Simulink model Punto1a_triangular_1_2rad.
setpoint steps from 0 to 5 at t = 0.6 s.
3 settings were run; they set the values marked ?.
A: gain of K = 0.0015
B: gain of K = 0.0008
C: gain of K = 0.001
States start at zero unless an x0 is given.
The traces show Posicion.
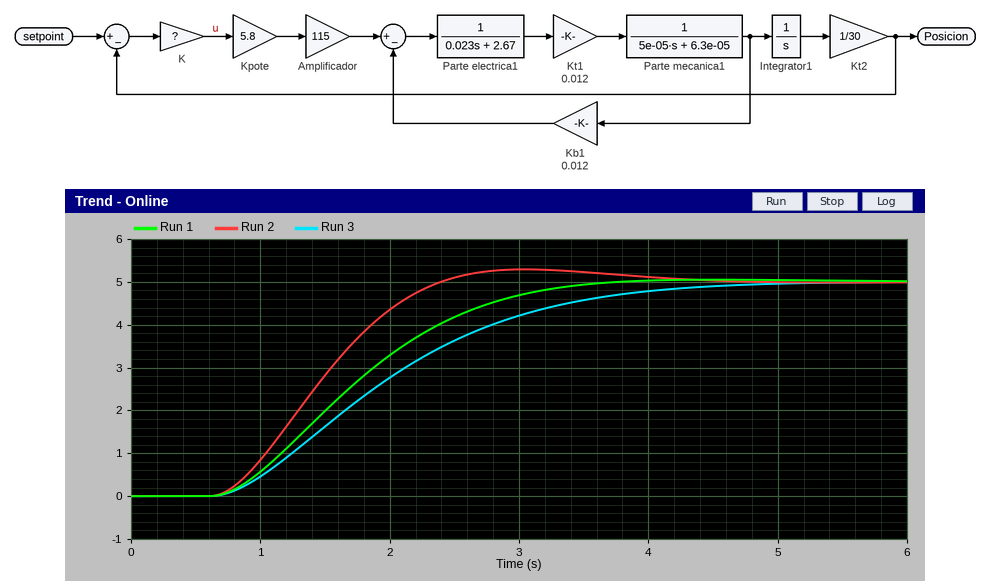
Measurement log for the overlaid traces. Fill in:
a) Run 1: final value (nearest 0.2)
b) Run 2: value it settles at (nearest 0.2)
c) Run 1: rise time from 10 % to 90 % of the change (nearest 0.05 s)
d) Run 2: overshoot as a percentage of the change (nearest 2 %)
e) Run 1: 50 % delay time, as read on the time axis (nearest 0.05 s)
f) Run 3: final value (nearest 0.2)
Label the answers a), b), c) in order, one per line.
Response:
a) 5.0
b) 5.0
c) 1.80 s
d) 6 %
e) 1.70 s
f) 5.0
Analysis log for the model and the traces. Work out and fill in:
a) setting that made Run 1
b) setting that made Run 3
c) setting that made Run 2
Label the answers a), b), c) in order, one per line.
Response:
a) C
b) B
c) A
